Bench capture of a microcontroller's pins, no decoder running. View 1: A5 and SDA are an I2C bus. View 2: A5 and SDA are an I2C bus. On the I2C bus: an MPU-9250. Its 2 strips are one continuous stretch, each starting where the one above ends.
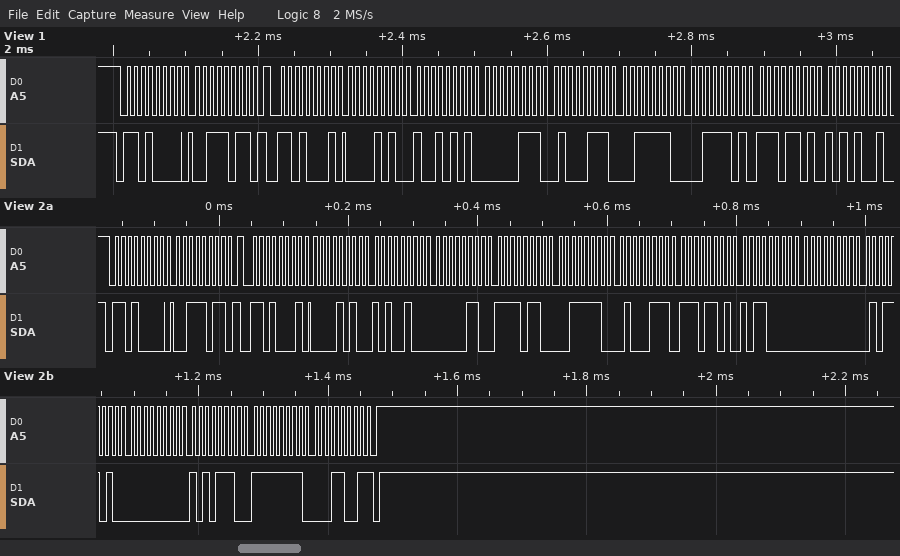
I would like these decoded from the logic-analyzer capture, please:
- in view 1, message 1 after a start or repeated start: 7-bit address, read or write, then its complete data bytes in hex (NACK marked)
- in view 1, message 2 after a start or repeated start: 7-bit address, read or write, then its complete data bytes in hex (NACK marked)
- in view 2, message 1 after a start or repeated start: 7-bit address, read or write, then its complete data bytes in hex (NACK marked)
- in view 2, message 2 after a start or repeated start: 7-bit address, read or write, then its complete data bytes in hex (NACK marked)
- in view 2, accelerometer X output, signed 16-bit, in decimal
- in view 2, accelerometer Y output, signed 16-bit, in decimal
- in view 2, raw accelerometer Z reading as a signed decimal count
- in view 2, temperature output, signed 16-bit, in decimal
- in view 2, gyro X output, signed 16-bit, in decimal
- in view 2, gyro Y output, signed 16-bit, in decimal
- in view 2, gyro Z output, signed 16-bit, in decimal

0x68 write: 3B
0x68 read: 0A 95 07 47 3E 3D ED A9
0x68 write: 3B
0x68 read: 0A A4 06 F6 3E 47 ED B0 00 5A 00 AE FF 19 NACK
2724
1782
15943
-4688
90
174
-231
